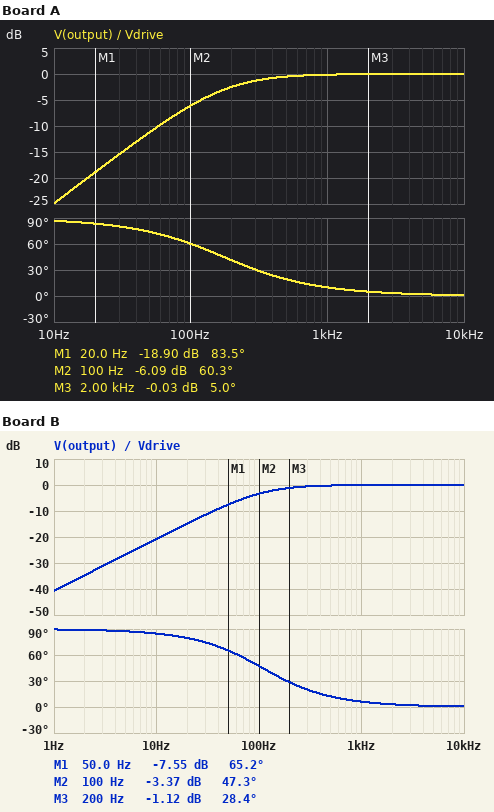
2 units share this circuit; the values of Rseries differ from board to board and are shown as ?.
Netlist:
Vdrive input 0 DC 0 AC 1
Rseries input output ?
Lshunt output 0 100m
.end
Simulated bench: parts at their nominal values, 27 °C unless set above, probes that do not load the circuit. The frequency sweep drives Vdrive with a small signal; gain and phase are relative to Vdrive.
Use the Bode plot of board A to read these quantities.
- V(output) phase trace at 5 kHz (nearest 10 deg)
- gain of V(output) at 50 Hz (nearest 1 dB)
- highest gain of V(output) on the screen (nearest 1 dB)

0 deg
-11 dB
0 dB
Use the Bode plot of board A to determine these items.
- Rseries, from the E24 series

110 Ω
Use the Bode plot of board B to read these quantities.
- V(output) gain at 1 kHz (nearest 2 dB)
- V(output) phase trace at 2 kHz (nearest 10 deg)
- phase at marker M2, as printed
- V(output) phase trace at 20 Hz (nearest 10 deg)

0 dB
0 deg
47.3 deg
80 deg
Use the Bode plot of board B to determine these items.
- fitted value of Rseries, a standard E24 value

68 Ω
